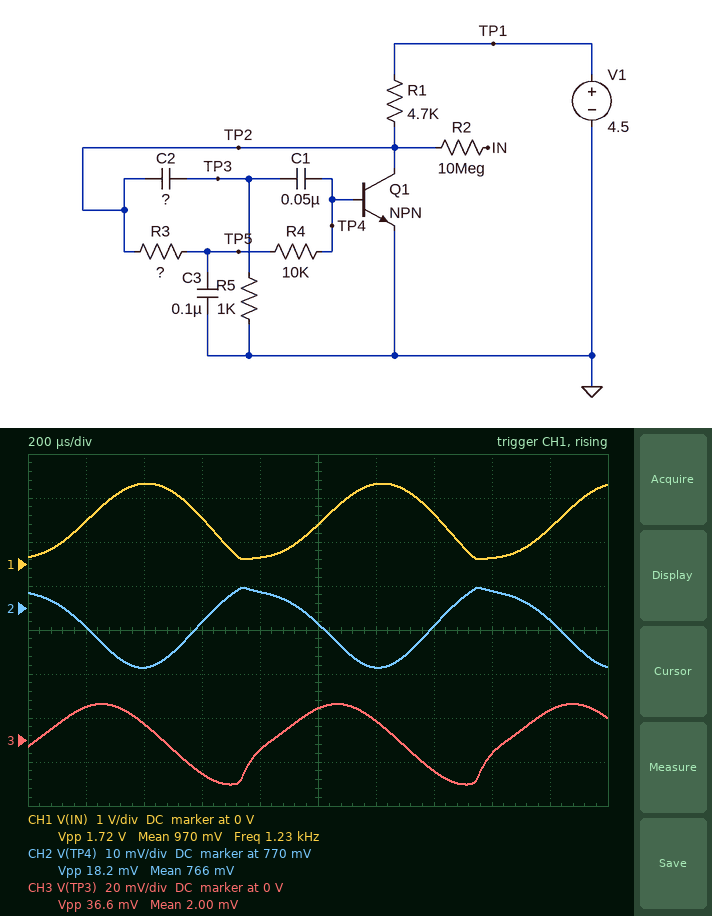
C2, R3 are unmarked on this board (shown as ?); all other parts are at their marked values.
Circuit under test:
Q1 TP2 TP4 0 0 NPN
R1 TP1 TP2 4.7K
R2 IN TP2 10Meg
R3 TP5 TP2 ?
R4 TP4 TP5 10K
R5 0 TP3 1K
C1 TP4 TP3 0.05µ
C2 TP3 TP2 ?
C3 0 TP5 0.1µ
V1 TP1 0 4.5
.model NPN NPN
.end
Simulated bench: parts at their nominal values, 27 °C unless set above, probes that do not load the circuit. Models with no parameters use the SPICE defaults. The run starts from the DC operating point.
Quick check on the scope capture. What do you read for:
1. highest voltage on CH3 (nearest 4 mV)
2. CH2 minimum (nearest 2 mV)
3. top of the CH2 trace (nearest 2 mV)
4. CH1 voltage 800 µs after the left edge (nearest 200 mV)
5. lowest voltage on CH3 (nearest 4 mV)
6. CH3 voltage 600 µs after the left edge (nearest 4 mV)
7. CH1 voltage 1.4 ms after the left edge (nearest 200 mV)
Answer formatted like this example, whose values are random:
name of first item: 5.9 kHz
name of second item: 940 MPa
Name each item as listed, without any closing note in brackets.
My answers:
highest voltage on CH3: 16 mV
CH2 minimum: 756 mV
top of the CH2 trace: 774 mV
CH1 voltage 800 µs after the left edge: 200 mV
lowest voltage on CH3: -20 mV
CH3 voltage 600 µs after the left edge: -16 mV
CH1 voltage 1.4 ms after the left edge: 1.2 V
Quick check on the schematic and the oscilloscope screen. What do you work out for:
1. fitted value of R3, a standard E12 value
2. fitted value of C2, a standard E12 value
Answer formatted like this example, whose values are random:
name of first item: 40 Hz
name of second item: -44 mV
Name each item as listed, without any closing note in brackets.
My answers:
fitted value of R3, a standard E12 value: 15 kΩ
fitted value of C2, a standard E12 value: 3.3 nF
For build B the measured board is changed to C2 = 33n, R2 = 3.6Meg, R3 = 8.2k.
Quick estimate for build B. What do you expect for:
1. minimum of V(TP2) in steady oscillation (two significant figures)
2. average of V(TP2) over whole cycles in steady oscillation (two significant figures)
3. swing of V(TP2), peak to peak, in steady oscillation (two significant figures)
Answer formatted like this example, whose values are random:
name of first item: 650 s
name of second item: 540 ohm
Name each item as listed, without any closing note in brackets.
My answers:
minimum of V(TP2) in steady oscillation: 65 mV
average of V(TP2) over whole cycles in steady oscillation: 1.0 V
swing of V(TP2), peak to peak, in steady oscillation: 2.0 V
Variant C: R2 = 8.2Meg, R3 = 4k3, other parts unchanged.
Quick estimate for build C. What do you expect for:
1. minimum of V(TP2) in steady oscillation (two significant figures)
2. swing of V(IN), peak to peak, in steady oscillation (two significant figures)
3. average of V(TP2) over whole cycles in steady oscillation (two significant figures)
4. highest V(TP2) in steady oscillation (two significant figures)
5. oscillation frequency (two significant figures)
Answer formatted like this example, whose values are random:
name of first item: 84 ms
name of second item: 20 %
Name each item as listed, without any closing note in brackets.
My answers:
minimum of V(TP2) in steady oscillation: 120 mV
swing of V(IN), peak to peak, in steady oscillation: 1.5 V
average of V(TP2) over whole cycles in steady oscillation: 890 mV
highest V(TP2) in steady oscillation: 1.6 V
oscillation frequency: 1.8 kHz
